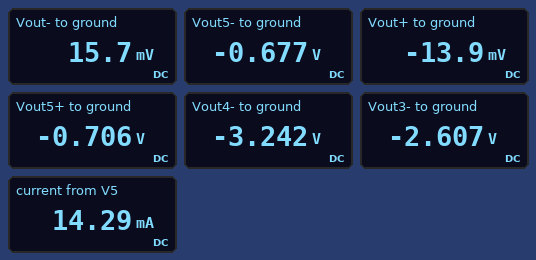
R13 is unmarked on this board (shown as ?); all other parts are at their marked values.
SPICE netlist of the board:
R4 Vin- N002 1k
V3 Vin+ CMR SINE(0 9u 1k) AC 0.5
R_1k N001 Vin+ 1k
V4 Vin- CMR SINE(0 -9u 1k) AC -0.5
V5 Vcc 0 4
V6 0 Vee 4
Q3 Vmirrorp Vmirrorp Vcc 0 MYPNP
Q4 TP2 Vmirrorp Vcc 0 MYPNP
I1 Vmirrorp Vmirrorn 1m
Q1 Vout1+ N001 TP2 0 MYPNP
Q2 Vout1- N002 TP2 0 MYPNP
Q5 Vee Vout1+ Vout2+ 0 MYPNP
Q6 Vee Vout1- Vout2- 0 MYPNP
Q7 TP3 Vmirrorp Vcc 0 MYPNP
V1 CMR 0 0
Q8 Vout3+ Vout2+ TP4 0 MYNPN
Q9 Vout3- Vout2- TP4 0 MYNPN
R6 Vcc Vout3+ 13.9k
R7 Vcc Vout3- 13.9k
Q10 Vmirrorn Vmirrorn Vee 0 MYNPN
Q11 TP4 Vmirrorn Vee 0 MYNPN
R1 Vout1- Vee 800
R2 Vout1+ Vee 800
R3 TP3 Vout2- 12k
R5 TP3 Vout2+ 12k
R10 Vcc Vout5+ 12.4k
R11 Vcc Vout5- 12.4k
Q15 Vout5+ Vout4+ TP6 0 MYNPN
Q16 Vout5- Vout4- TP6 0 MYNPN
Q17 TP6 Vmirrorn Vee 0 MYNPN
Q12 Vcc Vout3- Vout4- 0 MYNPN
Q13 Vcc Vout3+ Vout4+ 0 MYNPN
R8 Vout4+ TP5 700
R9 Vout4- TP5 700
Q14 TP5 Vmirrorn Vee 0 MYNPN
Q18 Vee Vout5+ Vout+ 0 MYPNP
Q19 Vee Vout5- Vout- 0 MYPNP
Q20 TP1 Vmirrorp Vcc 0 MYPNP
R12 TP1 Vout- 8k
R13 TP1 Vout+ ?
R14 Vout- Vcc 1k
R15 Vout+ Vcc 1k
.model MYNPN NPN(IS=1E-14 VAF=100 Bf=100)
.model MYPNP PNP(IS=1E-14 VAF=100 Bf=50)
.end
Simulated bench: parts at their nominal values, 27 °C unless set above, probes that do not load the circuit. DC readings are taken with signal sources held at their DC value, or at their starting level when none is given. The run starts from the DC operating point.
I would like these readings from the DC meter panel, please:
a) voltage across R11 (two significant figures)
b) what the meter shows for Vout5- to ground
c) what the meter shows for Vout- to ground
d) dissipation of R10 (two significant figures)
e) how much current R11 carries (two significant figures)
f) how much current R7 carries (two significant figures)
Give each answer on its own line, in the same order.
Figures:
4.7 V
-0.677 V
15.7 mV
1.8 mW
380 µA
480 µA
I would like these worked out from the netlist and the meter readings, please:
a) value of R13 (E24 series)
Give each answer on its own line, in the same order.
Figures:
12 kΩ
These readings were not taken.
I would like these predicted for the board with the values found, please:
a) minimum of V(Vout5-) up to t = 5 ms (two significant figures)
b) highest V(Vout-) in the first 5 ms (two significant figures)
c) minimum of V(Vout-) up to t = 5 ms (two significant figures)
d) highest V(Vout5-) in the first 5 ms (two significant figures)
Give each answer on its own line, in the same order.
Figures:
-3.2 V
2.5 V
-2.5 V
1.8 V
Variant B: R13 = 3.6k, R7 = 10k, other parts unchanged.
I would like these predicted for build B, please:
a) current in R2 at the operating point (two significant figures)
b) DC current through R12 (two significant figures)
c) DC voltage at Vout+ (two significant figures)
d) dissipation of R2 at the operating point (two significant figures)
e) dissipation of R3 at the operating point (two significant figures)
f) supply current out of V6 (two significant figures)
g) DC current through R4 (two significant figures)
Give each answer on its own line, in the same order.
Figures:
430 µA
680 µA
4.0 V
150 µW
2.2 mW
12 mA
8.2 µA
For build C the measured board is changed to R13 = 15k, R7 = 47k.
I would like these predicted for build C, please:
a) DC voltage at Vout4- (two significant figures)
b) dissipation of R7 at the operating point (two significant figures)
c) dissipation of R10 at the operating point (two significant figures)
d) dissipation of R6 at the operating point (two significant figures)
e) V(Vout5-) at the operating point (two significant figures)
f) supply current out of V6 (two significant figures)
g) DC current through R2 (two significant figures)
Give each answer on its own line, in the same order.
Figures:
-3.9 V
1.3 mW
640 µW
3.2 mW
4.0 V
6.3 mA
350 µA
